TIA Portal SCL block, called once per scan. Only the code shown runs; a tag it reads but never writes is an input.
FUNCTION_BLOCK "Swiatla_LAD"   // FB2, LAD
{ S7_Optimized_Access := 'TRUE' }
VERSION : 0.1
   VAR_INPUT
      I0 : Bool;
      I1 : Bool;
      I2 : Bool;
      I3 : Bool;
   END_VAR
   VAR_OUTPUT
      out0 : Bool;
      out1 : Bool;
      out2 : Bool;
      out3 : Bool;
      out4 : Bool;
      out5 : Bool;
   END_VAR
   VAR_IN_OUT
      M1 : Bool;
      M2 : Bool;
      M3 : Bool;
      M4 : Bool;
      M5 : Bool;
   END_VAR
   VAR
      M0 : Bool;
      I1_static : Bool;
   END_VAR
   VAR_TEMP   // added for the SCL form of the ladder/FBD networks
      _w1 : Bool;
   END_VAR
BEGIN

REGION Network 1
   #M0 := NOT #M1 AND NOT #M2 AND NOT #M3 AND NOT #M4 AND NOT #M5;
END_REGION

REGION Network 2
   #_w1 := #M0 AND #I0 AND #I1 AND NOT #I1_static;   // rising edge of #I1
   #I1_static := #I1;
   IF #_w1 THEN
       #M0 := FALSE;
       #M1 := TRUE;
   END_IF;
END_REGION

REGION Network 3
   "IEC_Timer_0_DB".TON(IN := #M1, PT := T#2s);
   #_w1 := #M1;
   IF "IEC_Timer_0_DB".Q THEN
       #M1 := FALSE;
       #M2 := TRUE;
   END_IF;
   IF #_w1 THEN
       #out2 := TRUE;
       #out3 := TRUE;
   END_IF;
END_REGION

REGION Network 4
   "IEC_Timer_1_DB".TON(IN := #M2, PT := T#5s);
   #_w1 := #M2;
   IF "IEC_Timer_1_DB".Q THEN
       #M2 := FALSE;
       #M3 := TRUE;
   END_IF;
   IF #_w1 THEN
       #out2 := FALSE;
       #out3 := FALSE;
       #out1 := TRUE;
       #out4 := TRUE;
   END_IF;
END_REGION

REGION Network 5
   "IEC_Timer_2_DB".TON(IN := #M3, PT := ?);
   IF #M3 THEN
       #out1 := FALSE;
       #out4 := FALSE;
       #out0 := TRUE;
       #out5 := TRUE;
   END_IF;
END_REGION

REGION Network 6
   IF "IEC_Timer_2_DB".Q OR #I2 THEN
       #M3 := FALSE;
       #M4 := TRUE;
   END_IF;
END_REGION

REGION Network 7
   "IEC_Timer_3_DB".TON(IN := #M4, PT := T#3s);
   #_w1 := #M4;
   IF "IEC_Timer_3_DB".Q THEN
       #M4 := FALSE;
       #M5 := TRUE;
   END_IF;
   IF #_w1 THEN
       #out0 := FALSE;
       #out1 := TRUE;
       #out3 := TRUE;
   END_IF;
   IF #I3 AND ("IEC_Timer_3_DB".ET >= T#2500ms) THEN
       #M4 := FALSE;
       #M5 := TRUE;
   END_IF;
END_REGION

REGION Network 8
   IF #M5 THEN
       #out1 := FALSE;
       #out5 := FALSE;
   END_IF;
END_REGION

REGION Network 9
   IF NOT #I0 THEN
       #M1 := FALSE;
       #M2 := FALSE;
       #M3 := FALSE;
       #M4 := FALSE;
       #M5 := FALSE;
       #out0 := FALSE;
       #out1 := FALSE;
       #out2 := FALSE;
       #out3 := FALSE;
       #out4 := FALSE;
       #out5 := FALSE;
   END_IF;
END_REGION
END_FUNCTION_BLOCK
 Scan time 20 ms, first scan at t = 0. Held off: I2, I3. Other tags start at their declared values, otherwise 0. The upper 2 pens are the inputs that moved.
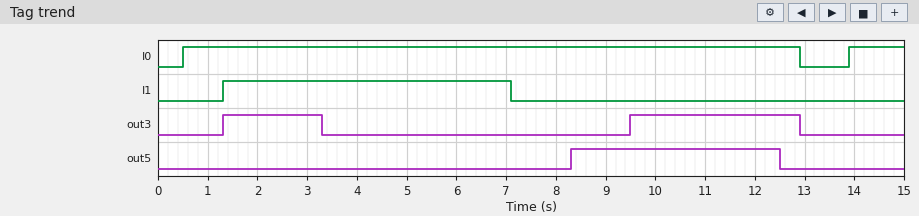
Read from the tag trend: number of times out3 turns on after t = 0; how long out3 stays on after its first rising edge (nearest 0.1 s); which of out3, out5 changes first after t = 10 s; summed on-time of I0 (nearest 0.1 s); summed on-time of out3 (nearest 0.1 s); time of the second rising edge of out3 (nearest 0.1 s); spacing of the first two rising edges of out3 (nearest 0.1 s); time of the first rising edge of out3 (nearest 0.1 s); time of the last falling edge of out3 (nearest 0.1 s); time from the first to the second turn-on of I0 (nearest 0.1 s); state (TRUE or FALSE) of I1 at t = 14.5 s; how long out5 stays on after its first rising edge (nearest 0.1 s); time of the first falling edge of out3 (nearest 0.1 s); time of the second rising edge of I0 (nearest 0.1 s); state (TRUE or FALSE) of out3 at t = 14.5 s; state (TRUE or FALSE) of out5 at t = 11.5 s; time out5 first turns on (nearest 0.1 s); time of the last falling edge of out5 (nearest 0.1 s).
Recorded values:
2
2.0 s
out5
13.5 s
5.4 s
9.5 s
8.2 s
1.3 s
12.9 s
13.4 s
FALSE
4.2 s
3.3 s
13.9 s
FALSE
TRUE
8.3 s
12.5 s
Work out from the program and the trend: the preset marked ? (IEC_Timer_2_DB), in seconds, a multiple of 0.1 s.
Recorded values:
1.2 s
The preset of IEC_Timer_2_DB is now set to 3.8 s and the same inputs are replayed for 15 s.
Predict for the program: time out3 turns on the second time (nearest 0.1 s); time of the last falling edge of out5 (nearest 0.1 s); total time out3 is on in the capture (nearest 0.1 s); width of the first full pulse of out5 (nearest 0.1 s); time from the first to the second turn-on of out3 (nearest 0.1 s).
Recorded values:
12.1 s
12.9 s
2.8 s
4.6 s
10.8 s
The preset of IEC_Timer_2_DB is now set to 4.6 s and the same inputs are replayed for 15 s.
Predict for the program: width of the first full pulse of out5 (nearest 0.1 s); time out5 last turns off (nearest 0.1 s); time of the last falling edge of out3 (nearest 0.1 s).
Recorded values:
4.6 s
12.9 s
3.3 s
